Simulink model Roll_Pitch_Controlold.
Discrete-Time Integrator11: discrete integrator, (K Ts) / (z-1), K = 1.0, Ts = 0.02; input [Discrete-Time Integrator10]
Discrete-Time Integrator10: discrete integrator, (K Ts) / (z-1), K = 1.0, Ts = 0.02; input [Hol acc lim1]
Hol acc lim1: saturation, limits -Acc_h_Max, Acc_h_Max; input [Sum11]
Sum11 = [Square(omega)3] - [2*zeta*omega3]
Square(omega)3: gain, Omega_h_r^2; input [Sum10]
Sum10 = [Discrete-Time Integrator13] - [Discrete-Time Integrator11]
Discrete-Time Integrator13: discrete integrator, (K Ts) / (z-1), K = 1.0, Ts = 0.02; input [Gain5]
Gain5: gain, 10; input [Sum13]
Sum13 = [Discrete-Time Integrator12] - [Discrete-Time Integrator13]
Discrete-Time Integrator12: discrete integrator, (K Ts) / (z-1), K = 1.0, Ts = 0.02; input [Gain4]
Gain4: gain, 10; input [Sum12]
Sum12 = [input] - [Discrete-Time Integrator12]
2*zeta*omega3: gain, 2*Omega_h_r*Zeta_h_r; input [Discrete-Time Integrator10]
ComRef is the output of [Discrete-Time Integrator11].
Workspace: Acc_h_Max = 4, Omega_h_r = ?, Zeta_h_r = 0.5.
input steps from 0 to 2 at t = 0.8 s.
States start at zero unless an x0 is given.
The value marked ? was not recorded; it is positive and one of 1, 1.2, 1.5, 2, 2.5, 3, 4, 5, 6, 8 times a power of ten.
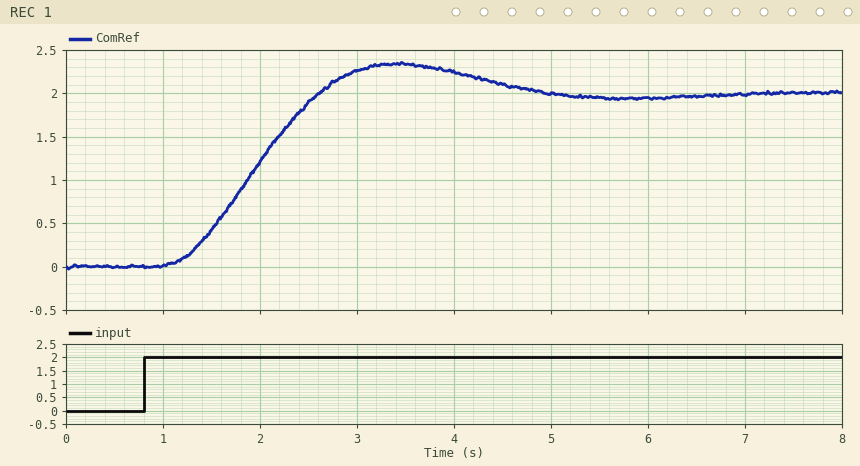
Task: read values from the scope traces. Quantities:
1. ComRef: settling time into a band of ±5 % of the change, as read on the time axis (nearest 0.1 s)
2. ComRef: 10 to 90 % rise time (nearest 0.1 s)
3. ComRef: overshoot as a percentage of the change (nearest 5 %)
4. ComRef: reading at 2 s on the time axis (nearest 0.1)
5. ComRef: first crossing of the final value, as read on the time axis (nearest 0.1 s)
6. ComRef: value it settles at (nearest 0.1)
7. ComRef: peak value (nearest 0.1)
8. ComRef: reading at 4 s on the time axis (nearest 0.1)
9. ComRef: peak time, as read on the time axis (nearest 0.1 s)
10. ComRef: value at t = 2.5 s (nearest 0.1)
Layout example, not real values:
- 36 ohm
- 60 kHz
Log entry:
- 4.5 s
- 1.1 s
- 15 %
- 1.2
- 2.6 s
- 2.0
- 2.3
- 2.2
- 3.4 s
- 1.9
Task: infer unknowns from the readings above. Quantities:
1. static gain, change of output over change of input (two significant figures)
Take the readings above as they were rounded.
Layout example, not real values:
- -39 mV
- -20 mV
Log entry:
- 1.0
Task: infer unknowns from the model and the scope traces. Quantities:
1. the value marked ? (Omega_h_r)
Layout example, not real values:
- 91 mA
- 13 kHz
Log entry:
- 1.5
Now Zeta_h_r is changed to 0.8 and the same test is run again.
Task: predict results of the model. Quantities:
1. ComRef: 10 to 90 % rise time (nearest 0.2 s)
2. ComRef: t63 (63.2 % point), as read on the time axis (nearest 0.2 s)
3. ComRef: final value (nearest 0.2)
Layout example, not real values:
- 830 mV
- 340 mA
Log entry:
- 1.6 s
- 2.2 s
- 2.0
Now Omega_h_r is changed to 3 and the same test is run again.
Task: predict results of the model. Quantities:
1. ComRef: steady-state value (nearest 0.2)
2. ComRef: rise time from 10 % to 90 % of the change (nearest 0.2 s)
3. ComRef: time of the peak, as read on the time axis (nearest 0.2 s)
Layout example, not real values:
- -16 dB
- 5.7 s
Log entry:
- 2.0
- 0.8 s
- 2.4 s
